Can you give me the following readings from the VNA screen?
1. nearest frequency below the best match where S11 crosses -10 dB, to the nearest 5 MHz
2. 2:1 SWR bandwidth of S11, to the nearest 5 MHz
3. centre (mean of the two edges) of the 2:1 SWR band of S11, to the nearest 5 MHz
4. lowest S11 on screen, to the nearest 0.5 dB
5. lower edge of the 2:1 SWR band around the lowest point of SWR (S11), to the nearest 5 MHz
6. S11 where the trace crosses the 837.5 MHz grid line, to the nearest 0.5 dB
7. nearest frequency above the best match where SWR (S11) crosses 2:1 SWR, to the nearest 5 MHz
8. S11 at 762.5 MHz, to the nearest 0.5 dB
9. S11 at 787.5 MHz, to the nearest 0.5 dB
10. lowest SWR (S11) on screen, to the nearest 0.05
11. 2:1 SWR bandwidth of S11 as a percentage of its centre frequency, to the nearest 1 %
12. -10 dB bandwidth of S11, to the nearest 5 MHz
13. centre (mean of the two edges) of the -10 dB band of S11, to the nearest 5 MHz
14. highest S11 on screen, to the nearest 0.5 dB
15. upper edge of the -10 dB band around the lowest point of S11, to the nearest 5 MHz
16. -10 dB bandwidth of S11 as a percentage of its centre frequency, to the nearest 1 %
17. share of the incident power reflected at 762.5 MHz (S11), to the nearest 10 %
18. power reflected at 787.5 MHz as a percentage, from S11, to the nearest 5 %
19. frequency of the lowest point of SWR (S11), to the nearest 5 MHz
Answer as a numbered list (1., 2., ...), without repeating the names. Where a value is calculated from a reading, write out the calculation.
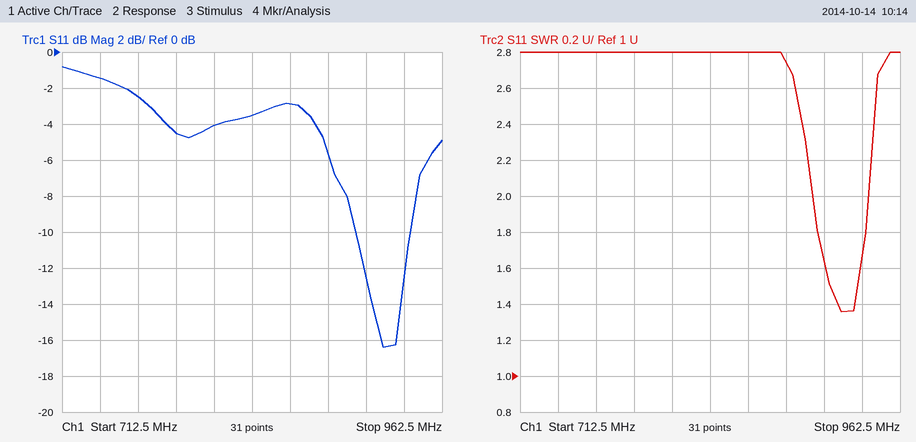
1. 905 MHz
2. 940 MHz − 905 MHz = 35 MHz
3. 925 MHz
4. -16.5 dB
5. 905 MHz
6. -3.5 dB
7. 940 MHz
8. -2.5 dB
9. -4.5 dB
10. 1.35
11. 35 MHz / 922.5 MHz ≈ 4 %
12. 940 MHz − 905 MHz = 35 MHz
13. 925 MHz
14. -1.0 dB
15. 940 MHz
16. 35 MHz / 922.5 MHz ≈ 4 %
17. 10^(-2.5/10) ≈ 56.2 %, so 60 % to the nearest 10 %
18. 10^(-4.5/10) ≈ 35 %
19. 925 MHz
